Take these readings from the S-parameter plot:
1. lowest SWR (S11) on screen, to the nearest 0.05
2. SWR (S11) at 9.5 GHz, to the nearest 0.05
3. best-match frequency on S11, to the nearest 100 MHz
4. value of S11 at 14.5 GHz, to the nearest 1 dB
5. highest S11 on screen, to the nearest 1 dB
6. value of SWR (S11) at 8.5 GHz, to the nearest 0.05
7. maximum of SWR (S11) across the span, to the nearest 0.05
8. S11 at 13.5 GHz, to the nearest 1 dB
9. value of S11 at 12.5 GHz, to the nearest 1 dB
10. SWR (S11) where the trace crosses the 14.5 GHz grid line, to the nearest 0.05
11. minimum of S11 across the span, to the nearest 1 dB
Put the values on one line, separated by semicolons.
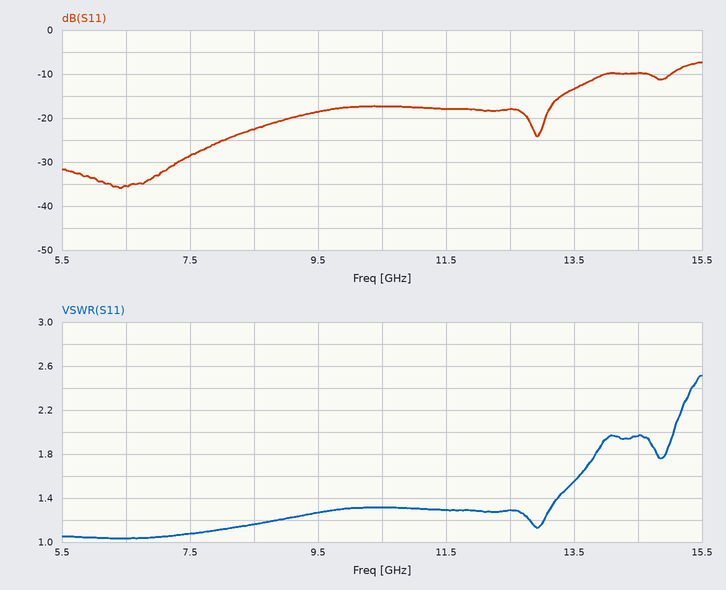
1.05; 1.25; 6.4 GHz; -10 dB; -7 dB; 1.15; 2.50; -13 dB; -18 dB; 1.95; -36 dB
